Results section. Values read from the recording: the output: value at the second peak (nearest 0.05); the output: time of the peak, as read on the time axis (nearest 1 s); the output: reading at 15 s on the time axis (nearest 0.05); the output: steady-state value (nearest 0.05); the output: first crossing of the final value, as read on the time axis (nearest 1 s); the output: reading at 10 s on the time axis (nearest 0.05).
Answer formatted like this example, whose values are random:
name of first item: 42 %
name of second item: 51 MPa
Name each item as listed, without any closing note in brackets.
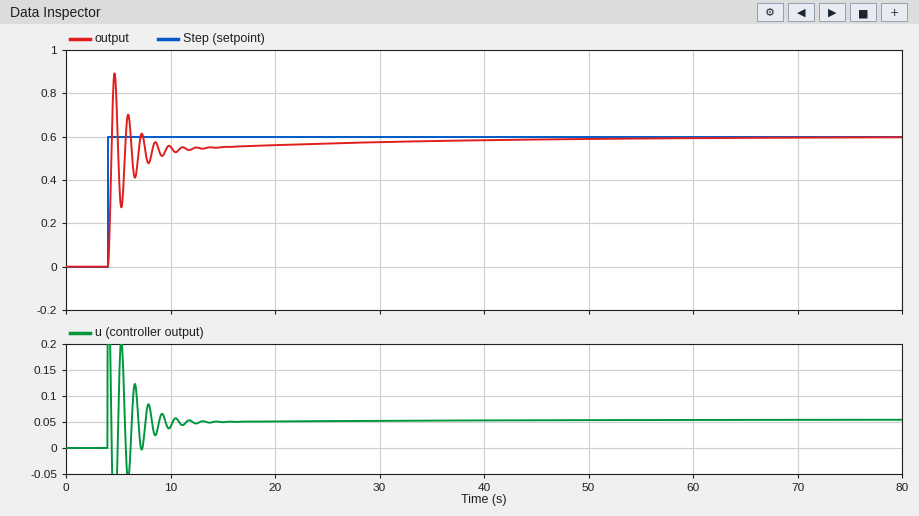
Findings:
the output: value at the second peak: 0.70
the output: time of the peak, as read on the time axis: 5 s
the output: reading at 15 s on the time axis: 0.55
the output: steady-state value: 0.60
the output: first crossing of the final value, as read on the time axis: 4 s
the output: reading at 10 s on the time axis: 0.55
